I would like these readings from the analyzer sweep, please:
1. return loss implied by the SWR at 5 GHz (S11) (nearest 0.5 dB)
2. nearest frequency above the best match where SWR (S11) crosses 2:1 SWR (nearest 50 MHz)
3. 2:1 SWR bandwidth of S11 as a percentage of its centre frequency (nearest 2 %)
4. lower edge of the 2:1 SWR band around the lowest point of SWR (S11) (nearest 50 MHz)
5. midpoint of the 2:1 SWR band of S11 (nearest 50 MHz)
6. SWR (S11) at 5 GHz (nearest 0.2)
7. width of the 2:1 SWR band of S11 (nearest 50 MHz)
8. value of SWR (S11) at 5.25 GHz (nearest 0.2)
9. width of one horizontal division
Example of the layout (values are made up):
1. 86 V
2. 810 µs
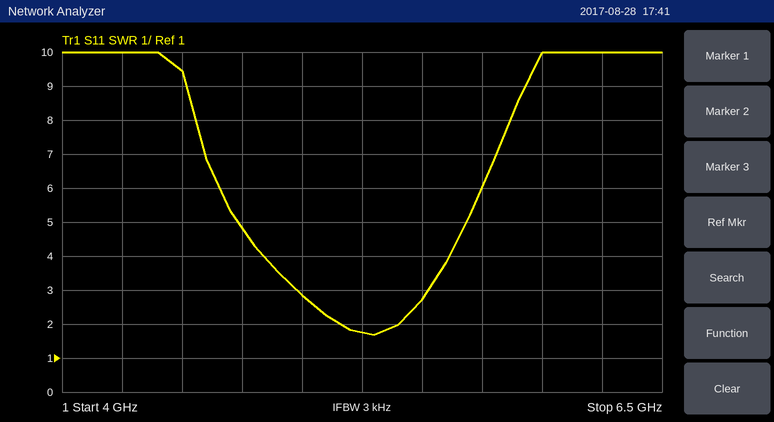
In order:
1. 6.5 dB
2. 5.40 GHz
3. 4 %
4. 5.15 GHz
5. 5.30 GHz
6. 2.8
7. 250 MHz
8. 1.8
9. 250 MHz
